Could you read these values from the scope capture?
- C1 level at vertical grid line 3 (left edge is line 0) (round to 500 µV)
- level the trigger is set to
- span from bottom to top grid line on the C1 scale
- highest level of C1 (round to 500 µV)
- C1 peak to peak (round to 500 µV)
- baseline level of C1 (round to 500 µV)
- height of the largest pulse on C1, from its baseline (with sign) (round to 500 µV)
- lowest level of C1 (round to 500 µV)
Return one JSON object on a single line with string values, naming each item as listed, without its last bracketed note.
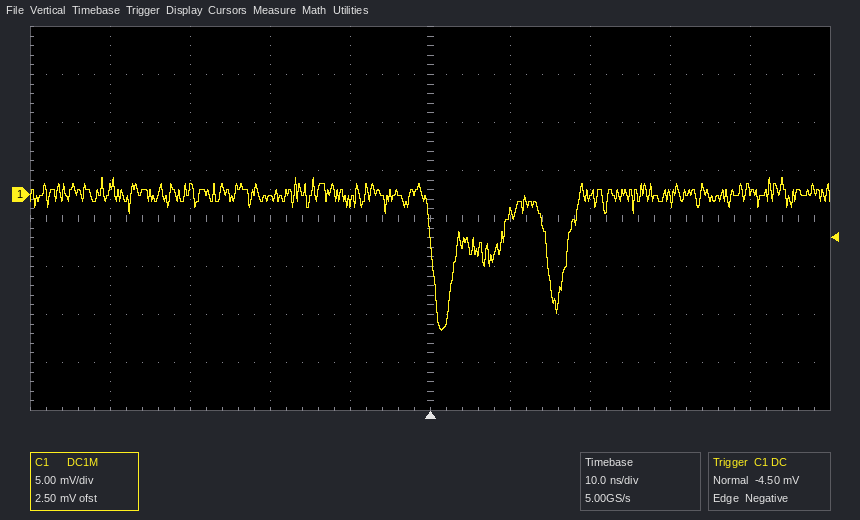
{"C1 level at vertical grid line 3 (left edge is line 0)": "-500 µV", "level the trigger is set to": "-4.50 mV", "span from bottom to top grid line on the C1 scale": "40 mV", "highest level of C1": "2.0 mV", "C1 peak to peak": "16.0 mV", "baseline level of C1": "0.0 mV", "height of the largest pulse on C1, from its baseline (with sign)": "-14.0 mV", "lowest level of C1": "-14.0 mV"}
